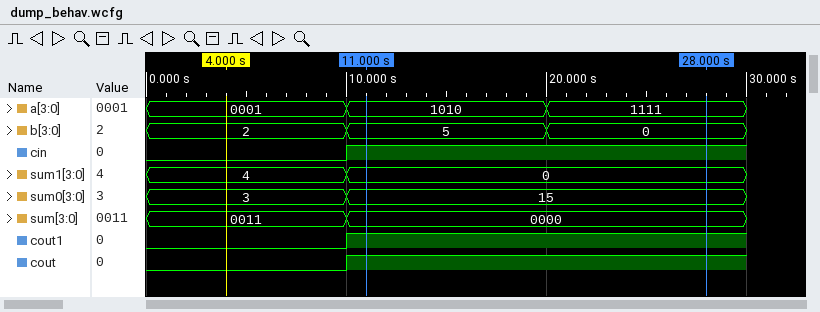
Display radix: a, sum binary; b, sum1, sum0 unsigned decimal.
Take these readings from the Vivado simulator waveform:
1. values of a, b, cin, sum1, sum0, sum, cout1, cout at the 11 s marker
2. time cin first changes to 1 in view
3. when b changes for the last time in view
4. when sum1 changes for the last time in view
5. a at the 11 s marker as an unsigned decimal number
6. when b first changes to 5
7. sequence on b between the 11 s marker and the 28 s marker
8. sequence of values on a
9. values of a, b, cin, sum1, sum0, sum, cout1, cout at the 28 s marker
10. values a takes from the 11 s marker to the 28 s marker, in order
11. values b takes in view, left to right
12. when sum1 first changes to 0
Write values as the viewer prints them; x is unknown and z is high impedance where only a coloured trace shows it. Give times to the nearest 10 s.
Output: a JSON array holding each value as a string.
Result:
["a=1010, b=5, cin=1, sum1=0, sum0=15, sum=0000, cout1=1, cout=1", "10 s", "20 s", "10 s", "10", "10 s", "5, 0", "0001, 1010, 1111", "a=1111, b=0, cin=1, sum1=0, sum0=15, sum=0000, cout1=1, cout=1", "1010, 1111", "2, 5, 0", "10 s"]
